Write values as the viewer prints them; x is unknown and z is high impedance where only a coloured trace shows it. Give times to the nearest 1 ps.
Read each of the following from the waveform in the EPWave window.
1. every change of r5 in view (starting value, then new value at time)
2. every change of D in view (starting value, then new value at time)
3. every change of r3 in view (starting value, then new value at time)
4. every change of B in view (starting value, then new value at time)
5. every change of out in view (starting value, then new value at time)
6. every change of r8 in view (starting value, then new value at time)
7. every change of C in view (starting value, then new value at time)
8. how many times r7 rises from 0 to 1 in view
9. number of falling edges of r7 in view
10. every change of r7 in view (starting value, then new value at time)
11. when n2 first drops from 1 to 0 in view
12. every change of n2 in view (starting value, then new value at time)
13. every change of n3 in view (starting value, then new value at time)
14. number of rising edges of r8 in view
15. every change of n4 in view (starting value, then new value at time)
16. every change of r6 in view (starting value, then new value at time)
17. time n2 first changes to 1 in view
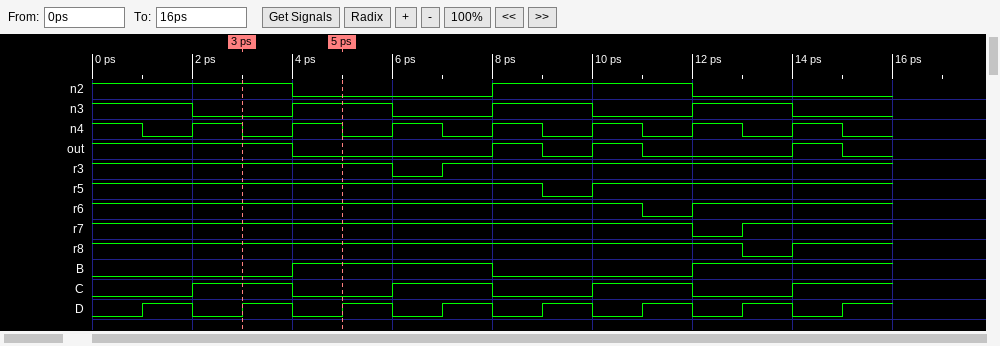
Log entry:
1, 0 at 9 ps, 1 at 10 ps
0, 1 at 1 ps, 0 at 2 ps, 1 at 3 ps, 0 at 4 ps, 1 at 5 ps, 0 at 6 ps, 1 at 7 ps, 0 at 8 ps, 1 at 9 ps, 0 at 10 ps, 1 at 11 ps, 0 at 12 ps, 1 at 13 ps, 0 at 14 ps, 1 at 15 ps
1, 0 at 6 ps, 1 at 7 ps
0, 1 at 4 ps, 0 at 8 ps, 1 at 12 ps
1, 0 at 4 ps, 1 at 8 ps, 0 at 9 ps, 1 at 10 ps, 0 at 11 ps, 1 at 14 ps, 0 at 15 ps
1, 0 at 13 ps, 1 at 14 ps
0, 1 at 2 ps, 0 at 4 ps, 1 at 6 ps, 0 at 8 ps, 1 at 10 ps, 0 at 12 ps, 1 at 14 ps
1
1
1, 0 at 12 ps, 1 at 13 ps
4 ps
1, 0 at 4 ps, 1 at 8 ps, 0 at 12 ps
1, 0 at 2 ps, 1 at 4 ps, 0 at 6 ps, 1 at 8 ps, 0 at 10 ps, 1 at 12 ps, 0 at 14 ps
1
1, 0 at 1 ps, 1 at 2 ps, 0 at 3 ps, 1 at 4 ps, 0 at 5 ps, 1 at 6 ps, 0 at 7 ps, 1 at 8 ps, 0 at 9 ps, 1 at 10 ps, 0 at 11 ps, 1 at 12 ps, 0 at 13 ps, 1 at 14 ps, 0 at 15 ps
1, 0 at 11 ps, 1 at 12 ps
8 ps
